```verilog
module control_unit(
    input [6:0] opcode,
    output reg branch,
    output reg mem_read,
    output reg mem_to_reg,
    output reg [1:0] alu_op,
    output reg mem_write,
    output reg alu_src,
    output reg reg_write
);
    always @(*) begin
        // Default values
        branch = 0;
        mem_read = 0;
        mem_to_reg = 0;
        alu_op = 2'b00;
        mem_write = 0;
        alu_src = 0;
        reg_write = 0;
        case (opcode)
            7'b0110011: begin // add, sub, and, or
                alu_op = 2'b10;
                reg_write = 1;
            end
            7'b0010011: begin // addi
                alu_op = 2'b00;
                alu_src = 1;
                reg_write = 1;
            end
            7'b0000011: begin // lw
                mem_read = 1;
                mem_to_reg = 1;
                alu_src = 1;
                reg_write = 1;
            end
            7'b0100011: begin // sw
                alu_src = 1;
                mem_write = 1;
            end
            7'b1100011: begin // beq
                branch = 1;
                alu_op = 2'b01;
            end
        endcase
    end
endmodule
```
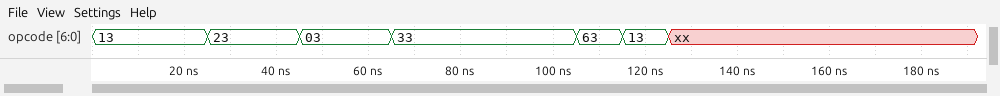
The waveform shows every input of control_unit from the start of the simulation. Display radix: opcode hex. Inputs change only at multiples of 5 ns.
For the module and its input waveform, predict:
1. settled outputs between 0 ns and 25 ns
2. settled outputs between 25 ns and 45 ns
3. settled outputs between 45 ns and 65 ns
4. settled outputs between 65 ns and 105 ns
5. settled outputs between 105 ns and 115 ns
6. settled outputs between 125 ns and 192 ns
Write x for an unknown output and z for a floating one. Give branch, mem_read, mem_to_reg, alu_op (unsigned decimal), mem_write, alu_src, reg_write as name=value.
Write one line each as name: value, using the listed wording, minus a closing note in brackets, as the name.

settled outputs between 0 ns and 25 ns: branch=0, mem_read=0, mem_to_reg=0, alu_op=0, mem_write=0, alu_src=1, reg_write=1
settled outputs between 25 ns and 45 ns: branch=0, mem_read=0, mem_to_reg=0, alu_op=0, mem_write=1, alu_src=1, reg_write=0
settled outputs between 45 ns and 65 ns: branch=0, mem_read=1, mem_to_reg=1, alu_op=0, mem_write=0, alu_src=1, reg_write=1
settled outputs between 65 ns and 105 ns: branch=0, mem_read=0, mem_to_reg=0, alu_op=2, mem_write=0, alu_src=0, reg_write=1
settled outputs between 105 ns and 115 ns: branch=1, mem_read=0, mem_to_reg=0, alu_op=1, mem_write=0, alu_src=0, reg_write=0
settled outputs between 125 ns and 192 ns: branch=0, mem_read=0, mem_to_reg=0, alu_op=0, mem_write=0, alu_src=0, reg_write=0
